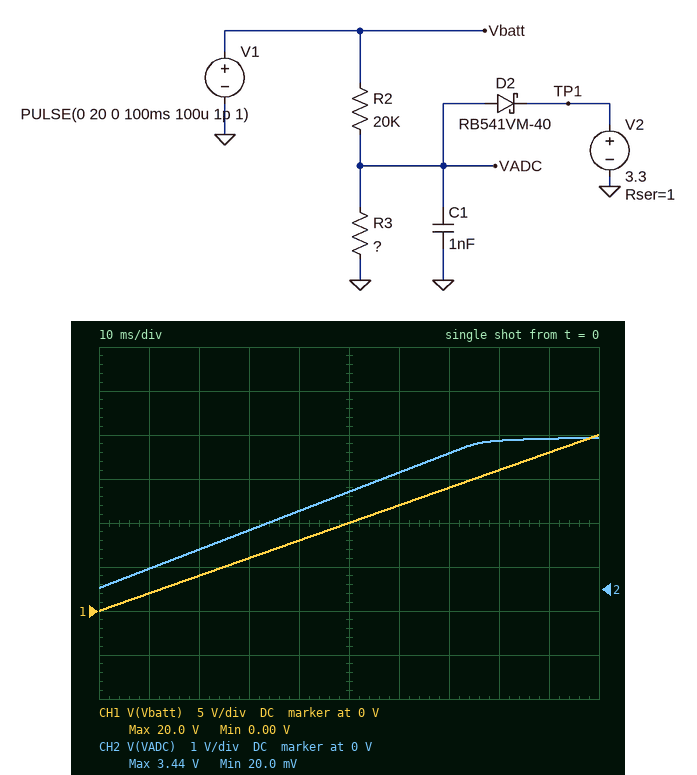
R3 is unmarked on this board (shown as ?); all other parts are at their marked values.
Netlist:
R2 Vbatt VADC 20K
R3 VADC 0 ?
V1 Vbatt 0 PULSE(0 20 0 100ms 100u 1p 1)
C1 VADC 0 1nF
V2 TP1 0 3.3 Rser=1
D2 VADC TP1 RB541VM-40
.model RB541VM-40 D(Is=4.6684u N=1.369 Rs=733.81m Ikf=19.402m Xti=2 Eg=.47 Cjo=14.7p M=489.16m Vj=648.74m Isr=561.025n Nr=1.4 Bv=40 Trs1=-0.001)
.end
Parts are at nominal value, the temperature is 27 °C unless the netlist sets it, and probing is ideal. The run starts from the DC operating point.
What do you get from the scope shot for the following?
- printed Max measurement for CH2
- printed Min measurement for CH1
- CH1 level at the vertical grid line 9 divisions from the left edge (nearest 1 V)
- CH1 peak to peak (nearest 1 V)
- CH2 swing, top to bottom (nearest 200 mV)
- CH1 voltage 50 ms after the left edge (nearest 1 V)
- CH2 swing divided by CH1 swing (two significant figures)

3.44 V
0.00 V
18 V
20 V
3.4 V
10 V
0.17
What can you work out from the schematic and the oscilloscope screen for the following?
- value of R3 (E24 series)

5.6 kΩ
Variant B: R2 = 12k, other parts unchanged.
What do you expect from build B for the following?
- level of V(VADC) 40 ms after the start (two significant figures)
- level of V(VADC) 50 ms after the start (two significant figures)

2.6 V
3.2 V
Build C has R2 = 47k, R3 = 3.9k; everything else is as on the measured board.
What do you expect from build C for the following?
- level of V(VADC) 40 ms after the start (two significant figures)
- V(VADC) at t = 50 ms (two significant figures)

630 mV
780 mV
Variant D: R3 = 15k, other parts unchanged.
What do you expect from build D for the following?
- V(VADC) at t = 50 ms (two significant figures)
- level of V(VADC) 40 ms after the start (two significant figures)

3.4 V
3.3 V
